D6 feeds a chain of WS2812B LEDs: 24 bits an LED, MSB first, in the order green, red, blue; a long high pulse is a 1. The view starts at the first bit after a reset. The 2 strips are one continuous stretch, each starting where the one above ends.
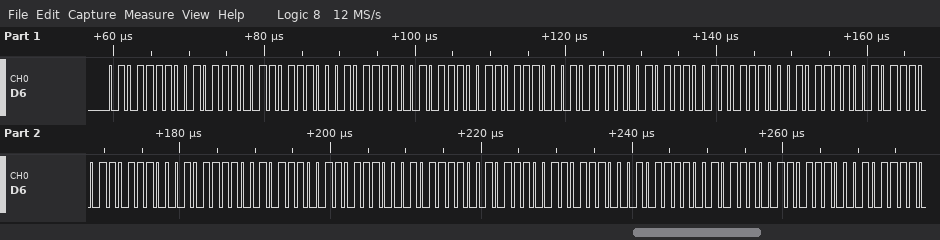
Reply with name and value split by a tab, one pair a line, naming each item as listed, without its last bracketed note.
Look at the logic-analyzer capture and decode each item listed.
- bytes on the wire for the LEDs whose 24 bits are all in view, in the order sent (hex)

bytes on the wire for the LEDs whose 24 bits are all in view, in the order sent	5E 5C DC 5E 5C DC 5E 5C DC 5E 5C DC 5E 5C DC 5E 5C DC 5E 5C DC
